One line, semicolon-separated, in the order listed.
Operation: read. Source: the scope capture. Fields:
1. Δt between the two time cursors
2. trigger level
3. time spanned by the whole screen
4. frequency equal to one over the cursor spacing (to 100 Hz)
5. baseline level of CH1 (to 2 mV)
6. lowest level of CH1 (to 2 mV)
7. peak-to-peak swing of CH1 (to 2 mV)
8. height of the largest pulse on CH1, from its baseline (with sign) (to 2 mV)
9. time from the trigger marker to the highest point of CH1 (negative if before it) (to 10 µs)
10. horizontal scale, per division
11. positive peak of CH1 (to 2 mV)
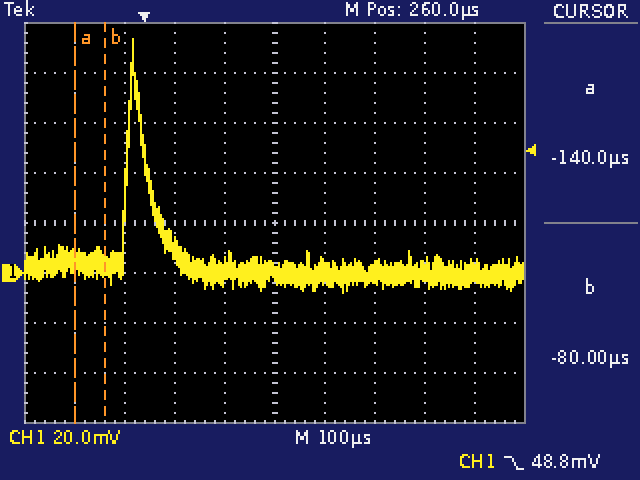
60 µs; 48.8 mV; 1 ms; 16.7 kHz; 0 mV; -8 mV; 102 mV; +94 mV; -20 µs; 100 µs; 94 mV
